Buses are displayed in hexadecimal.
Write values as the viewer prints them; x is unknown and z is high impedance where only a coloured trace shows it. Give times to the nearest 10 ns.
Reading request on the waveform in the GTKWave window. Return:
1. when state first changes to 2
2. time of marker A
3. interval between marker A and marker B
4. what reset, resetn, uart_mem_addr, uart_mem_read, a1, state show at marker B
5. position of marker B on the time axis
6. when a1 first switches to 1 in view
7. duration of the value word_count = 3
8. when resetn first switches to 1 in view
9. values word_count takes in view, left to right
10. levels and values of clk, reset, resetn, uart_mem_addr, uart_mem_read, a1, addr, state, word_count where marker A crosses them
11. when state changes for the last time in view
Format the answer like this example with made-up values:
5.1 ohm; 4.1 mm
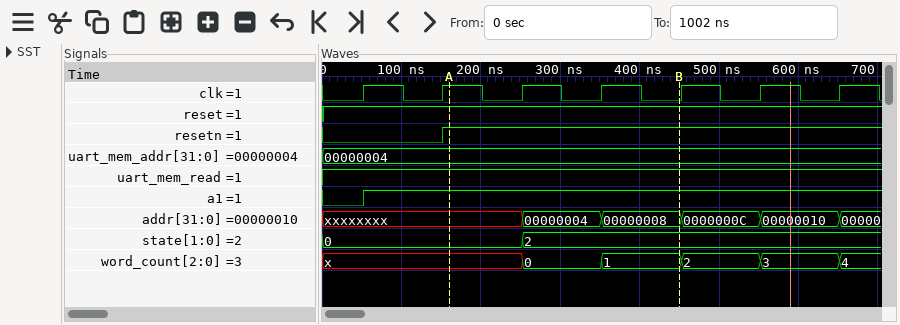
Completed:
250 ns; 160 ns; 290 ns; reset=1, resetn=1, uart_mem_addr=00000004, uart_mem_read=1, a1=1, state=2; 450 ns; 50 ns; 100 ns; 150 ns; x, 0, 1, 2, 3, 4; clk=1, reset=1, resetn=1, uart_mem_addr=00000004, uart_mem_read=1, a1=1, addr=xxxxxxxx, state=0, word_count=x; 250 ns
